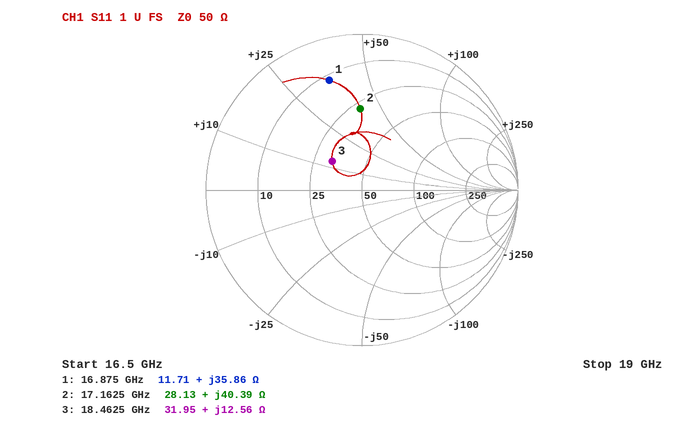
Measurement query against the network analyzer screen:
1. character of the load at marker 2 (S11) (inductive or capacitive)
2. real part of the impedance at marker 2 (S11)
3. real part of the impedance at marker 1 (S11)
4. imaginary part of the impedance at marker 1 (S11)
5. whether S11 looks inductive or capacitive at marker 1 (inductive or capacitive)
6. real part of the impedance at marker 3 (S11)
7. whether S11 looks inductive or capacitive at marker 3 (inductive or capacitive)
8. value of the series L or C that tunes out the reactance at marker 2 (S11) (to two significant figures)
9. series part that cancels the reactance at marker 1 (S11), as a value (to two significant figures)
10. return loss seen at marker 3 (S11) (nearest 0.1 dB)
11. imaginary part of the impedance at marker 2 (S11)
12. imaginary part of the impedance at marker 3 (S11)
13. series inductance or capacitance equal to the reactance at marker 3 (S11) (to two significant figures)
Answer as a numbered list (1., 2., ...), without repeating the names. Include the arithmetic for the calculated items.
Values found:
1. inductive
2. 28.13 Ω
3. 11.71 Ω
4. +35.86 Ω
5. inductive
6. 31.95 Ω
7. inductive
8. C = 1/(2π × 17.1625 GHz × 40.39 Ω) ≈ 230 fF
9. C = 1/(2π × 16.875 GHz × 35.86 Ω) ≈ 263 fF, so 260 fF to two significant figures
10. 11.5 dB
11. +40.39 Ω
12. +12.56 Ω
13. L = 12.56 Ω/(2π × 18.4625 GHz) ≈ 108 pH, so 110 pH to two significant figures
